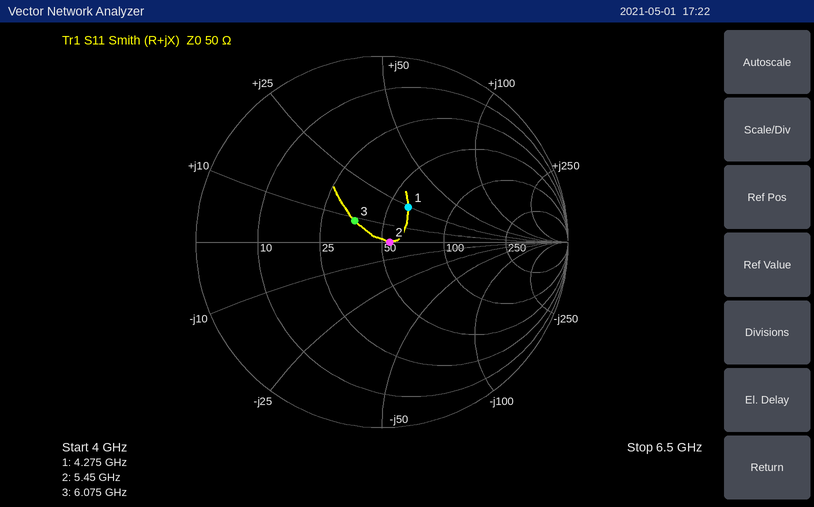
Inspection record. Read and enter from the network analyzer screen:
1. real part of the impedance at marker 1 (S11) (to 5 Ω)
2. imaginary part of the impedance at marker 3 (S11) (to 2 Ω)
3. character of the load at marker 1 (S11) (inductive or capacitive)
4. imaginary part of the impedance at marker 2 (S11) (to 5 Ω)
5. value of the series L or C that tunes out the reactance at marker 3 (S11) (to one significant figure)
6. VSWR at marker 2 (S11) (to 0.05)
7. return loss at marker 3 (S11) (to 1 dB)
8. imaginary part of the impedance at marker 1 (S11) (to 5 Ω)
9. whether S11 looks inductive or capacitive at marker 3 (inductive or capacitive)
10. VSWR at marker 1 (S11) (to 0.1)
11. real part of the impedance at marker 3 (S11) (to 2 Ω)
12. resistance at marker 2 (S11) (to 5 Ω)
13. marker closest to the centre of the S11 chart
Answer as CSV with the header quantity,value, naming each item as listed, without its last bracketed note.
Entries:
quantity,value
real part of the impedance at marker 1 (S11),60 Ω
imaginary part of the impedance at marker 3 (S11),+8 Ω
character of the load at marker 1 (S11),inductive
imaginary part of the impedance at marker 2 (S11),0 Ω
value of the series L or C that tunes out the reactance at marker 3 (S11),3 pF
VSWR at marker 2 (S11),1.10
return loss at marker 3 (S11),15 dB
imaginary part of the impedance at marker 1 (S11),+25 Ω
whether S11 looks inductive or capacitive at marker 3,inductive
VSWR at marker 1 (S11),1.6
real part of the impedance at marker 3 (S11),36 Ω
resistance at marker 2 (S11),55 Ω
marker closest to the centre of the S11 chart,marker 2
